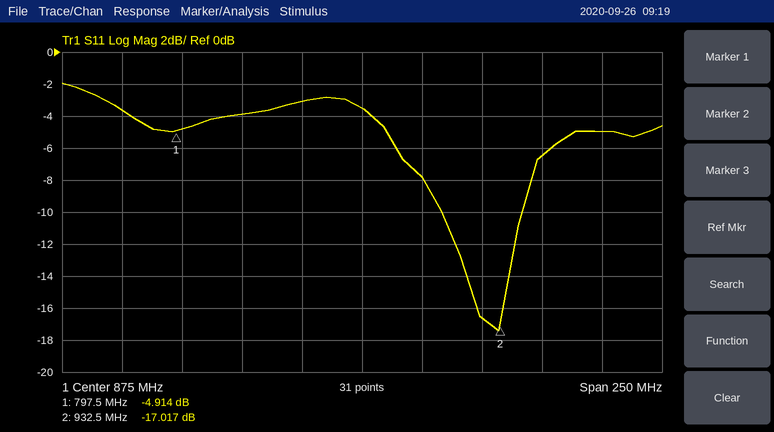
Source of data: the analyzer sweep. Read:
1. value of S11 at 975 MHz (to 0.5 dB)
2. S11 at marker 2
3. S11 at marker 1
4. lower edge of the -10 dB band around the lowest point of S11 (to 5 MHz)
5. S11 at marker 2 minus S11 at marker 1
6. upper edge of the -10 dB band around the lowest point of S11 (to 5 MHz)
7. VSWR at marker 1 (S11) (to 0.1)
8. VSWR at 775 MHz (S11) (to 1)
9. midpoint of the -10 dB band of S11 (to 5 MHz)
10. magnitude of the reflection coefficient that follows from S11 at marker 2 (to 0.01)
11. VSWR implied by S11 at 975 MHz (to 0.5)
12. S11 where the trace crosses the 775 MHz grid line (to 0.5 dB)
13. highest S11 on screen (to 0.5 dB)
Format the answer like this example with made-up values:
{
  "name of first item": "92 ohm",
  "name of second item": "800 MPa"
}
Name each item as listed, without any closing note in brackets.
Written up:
{
  "value of S11 at 975 MHz": "-5.0 dB",
  "S11 at marker 2": "-17.017 dB",
  "S11 at marker 1": "-4.914 dB",
  "lower edge of the -10 dB band around the lowest point of S11": "910 MHz",
  "S11 at marker 2 minus S11 at marker 1": "-12.103 dB",
  "upper edge of the -10 dB band around the lowest point of S11": "940 MHz",
  "VSWR at marker 1 (S11)": "3.6",
  "VSWR at 775 MHz (S11)": "5",
  "midpoint of the -10 dB band of S11": "925 MHz",
  "magnitude of the reflection coefficient that follows from S11 at marker 2": "0.14",
  "VSWR implied by S11 at 975 MHz": "3.5",
  "S11 where the trace crosses the 775 MHz grid line": "-3.5 dB",
  "highest S11 on screen": "-2.0 dB"
}
